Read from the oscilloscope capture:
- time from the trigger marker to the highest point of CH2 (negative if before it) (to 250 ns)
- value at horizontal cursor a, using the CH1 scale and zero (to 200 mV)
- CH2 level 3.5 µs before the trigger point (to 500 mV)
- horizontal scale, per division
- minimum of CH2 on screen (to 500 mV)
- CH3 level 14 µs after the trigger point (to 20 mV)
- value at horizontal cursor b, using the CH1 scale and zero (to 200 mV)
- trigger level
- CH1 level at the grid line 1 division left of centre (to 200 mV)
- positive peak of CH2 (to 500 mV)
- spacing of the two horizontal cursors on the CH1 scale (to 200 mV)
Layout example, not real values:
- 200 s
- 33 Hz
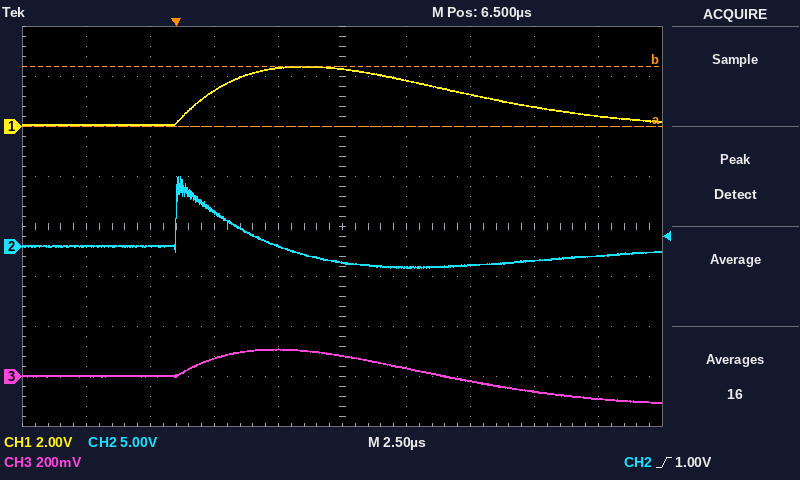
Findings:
- +250 ns
- 0.0 V
- 0.0 V
- 2.5 µs
- -2.0 V
- -60 mV
- 2.4 V
- 1.00 V
- 2.4 V
- 7.0 V
- 2.4 V
